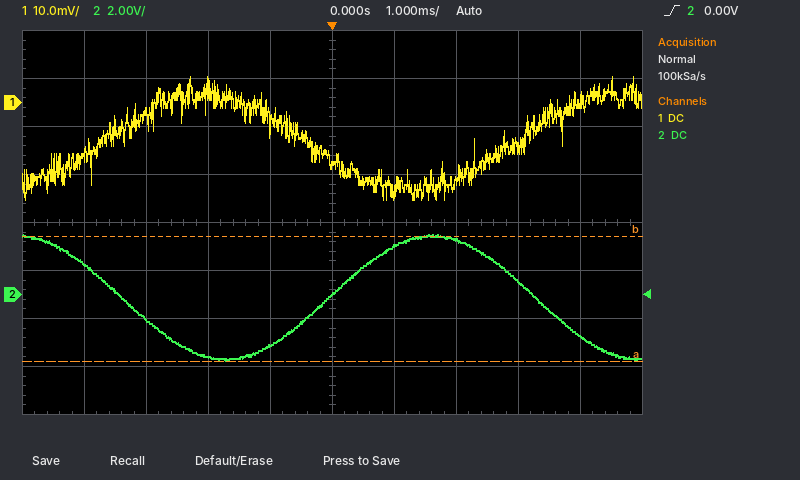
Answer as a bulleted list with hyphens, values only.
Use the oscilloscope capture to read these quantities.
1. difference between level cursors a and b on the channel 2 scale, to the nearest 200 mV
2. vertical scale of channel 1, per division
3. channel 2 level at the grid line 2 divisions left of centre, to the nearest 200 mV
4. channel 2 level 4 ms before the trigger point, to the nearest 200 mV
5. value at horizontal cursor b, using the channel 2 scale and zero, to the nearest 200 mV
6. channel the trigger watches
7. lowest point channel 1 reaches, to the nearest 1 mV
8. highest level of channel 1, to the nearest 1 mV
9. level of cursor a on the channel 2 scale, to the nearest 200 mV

- 5.2 V
- 10 mV
- -2.6 V
- 1.2 V
- 2.4 V
- channel 2
- -20 mV
- 5 mV
- -2.8 V
